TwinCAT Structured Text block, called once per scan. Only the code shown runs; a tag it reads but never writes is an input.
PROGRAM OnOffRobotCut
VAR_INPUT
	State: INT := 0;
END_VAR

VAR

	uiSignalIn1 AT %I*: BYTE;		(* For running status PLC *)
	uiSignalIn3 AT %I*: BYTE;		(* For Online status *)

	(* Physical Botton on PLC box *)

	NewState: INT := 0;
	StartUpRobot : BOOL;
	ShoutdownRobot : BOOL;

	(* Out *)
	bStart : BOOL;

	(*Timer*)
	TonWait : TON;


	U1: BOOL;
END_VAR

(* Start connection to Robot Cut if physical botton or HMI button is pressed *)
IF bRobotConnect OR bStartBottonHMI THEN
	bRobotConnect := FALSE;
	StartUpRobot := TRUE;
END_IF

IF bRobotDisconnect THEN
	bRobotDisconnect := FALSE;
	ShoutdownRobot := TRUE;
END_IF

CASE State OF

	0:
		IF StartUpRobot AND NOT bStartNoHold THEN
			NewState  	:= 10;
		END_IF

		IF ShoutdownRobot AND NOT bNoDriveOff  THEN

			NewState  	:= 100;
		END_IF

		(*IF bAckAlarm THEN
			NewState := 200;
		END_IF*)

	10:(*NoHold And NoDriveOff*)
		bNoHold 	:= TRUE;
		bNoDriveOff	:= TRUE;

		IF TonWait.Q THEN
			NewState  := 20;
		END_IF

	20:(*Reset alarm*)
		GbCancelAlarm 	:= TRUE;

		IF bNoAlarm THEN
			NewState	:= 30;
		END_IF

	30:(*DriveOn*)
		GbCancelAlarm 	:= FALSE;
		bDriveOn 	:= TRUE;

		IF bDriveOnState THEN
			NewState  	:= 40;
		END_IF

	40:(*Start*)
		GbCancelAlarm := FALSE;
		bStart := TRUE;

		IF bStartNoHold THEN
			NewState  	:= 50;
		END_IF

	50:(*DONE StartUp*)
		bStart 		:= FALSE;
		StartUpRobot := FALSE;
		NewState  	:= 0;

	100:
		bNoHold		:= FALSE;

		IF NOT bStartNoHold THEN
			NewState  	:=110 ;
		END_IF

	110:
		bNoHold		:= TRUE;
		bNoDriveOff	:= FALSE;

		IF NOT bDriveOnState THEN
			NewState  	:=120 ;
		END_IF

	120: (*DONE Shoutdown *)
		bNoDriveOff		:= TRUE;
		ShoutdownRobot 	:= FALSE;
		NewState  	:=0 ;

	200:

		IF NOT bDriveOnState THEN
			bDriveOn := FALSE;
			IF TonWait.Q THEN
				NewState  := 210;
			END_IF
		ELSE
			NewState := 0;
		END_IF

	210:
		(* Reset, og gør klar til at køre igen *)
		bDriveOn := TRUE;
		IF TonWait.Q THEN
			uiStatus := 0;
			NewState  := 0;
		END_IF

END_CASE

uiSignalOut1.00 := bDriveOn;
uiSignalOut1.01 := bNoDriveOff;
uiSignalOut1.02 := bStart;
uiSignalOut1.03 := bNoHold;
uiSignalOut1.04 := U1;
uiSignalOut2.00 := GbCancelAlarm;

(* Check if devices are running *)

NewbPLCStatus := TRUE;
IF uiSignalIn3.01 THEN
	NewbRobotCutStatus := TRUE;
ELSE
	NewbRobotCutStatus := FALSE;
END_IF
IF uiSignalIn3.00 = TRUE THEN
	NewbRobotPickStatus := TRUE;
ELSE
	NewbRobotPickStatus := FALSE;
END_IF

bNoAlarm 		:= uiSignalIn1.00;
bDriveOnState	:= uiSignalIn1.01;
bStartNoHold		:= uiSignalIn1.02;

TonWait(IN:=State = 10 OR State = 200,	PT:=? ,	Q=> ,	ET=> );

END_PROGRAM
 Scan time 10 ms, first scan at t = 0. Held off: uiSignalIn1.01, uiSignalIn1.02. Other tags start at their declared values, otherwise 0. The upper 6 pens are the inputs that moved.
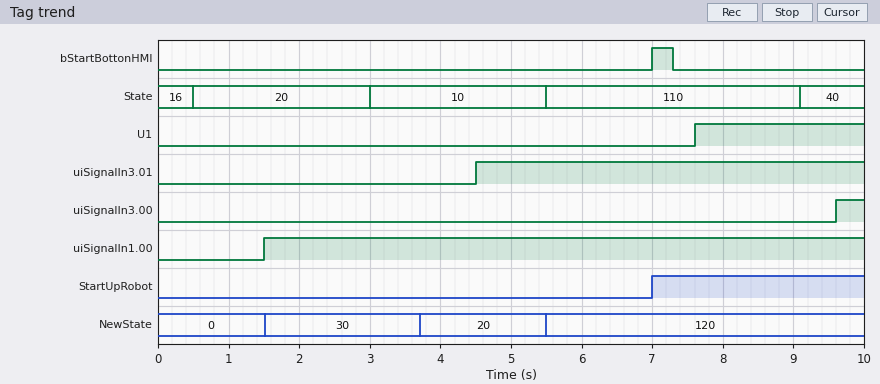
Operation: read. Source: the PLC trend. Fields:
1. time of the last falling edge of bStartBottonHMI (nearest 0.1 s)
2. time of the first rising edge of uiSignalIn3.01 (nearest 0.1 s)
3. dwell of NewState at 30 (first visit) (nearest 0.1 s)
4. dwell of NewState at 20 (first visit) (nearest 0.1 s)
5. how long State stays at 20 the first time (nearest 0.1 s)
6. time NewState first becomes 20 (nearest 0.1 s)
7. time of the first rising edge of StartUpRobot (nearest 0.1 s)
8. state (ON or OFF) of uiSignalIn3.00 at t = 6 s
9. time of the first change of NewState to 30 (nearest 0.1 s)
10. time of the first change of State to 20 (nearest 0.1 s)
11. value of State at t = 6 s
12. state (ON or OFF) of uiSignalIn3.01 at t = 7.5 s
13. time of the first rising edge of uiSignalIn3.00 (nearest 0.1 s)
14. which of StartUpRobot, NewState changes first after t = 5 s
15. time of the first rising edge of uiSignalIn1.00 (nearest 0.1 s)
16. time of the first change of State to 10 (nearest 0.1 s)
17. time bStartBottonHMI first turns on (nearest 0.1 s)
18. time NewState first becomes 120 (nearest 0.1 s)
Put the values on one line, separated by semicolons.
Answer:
7.3 s; 4.5 s; 2.2 s; 1.8 s; 2.5 s; 3.7 s; 7.0 s; OFF; 1.5 s; 0.5 s; 110; ON; 9.6 s; NewState; 1.5 s; 3.0 s; 7.0 s; 5.5 s
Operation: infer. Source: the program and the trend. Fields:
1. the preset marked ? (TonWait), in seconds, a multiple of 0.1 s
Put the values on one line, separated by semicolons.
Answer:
0.7 s
